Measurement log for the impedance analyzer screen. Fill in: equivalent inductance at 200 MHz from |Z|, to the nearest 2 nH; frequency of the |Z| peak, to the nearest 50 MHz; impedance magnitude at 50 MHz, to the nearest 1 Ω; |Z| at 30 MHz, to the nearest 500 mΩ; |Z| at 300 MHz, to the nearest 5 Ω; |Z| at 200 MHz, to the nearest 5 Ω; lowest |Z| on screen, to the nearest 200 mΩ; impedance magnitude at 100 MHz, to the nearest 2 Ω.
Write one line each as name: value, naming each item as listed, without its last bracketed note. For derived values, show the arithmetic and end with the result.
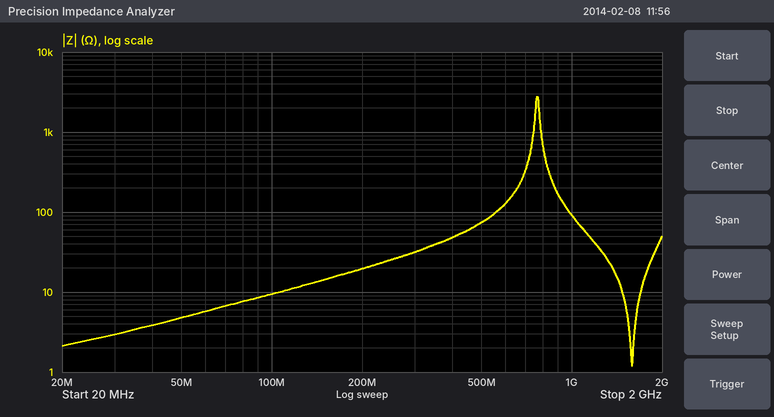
equivalent inductance at 200 MHz from |Z|, to the nearest 2 nH: L = 20 Ω/(2π × 200 MHz) ≈ 16 nH
frequency of the |Z| peak, to the nearest 50 MHz: 750 MHz
impedance magnitude at 50 MHz, to the nearest 1 Ω: 5 Ω
|Z| at 30 MHz, to the nearest 500 mΩ: 3.0 Ω
|Z| at 300 MHz, to the nearest 5 Ω: 30 Ω
|Z| at 200 MHz, to the nearest 5 Ω: 20 Ω
lowest |Z| on screen, to the nearest 200 mΩ: 1.2 Ω
impedance magnitude at 100 MHz, to the nearest 2 Ω: 10 Ω
